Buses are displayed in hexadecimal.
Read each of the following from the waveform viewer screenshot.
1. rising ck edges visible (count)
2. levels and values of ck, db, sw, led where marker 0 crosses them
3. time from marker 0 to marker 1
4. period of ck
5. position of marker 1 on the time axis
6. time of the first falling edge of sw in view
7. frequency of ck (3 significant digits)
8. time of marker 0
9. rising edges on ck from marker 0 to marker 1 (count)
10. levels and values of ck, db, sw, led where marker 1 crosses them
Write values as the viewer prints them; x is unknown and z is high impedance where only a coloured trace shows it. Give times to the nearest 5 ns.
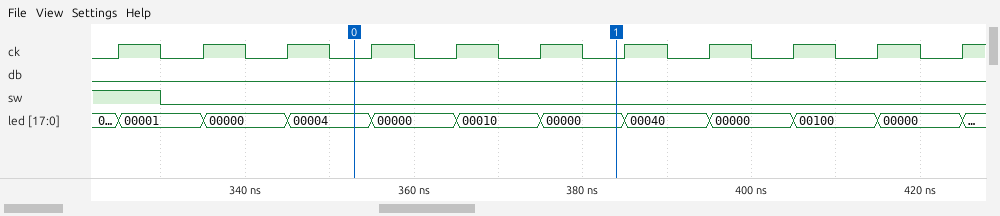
11
ck=0, db=0, sw=0, led=00004
30 ns
10 ns
385 ns
330 ns
100 MHz
355 ns
3
ck=0, db=0, sw=0, led=00000
